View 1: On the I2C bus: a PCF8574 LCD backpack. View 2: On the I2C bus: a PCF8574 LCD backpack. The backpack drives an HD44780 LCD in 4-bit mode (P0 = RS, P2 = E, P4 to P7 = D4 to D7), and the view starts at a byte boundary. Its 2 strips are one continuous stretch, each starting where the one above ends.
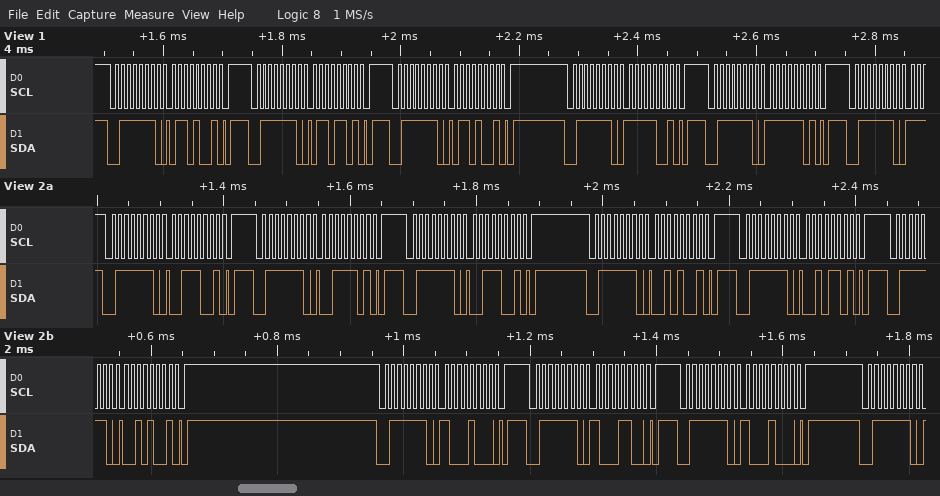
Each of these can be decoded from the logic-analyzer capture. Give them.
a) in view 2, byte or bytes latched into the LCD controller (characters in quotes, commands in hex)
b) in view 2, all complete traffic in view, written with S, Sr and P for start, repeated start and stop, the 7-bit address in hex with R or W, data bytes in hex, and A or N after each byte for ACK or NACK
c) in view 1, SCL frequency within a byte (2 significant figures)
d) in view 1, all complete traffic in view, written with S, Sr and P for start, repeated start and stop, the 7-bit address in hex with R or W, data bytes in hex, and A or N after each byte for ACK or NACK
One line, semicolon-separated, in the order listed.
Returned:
'2'; S 3FW A 39 A P S 3FW A 3D A P S 3FW A 39 A P S 3FW A 29 A P S 3FW A 2D A P S 3FW A 29 A P S 3FW A 88 A P S 3FW A 8C A P S 3FW A 88 A P S 3FW A; 100 kHz; S 3FW A 69 A P S 3FW A 6D A P S 3FW A 69 A P S 3FW A F9 A P S 3FW A FD A P S 3FW A
